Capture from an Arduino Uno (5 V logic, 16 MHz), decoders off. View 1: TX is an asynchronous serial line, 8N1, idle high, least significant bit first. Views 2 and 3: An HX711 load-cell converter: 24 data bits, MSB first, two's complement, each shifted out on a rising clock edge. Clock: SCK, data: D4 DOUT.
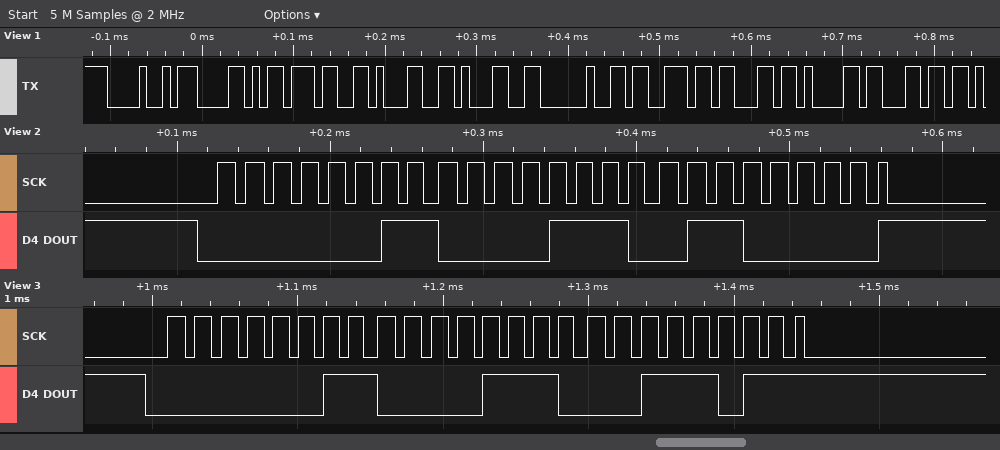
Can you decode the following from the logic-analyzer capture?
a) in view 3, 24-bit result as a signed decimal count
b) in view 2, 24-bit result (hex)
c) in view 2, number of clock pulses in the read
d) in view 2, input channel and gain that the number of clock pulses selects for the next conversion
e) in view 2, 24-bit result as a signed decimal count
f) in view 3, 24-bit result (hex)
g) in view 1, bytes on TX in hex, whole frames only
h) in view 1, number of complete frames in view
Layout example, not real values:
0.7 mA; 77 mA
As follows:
200251; 0x030E60; 25; channel A, gain 128; 200288; 0x030E3B; 48 58 37 31 31 20 73 63 61 6C; 10
